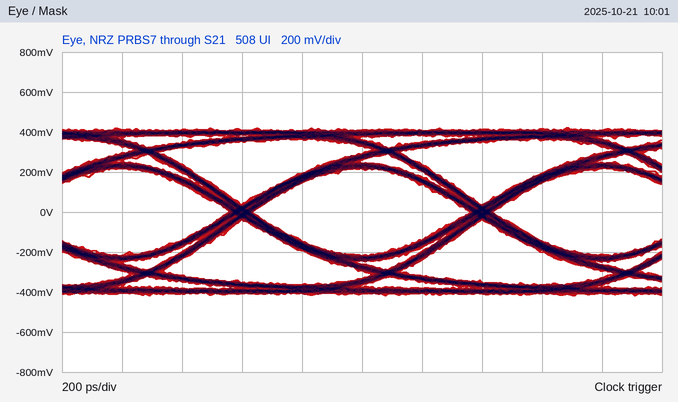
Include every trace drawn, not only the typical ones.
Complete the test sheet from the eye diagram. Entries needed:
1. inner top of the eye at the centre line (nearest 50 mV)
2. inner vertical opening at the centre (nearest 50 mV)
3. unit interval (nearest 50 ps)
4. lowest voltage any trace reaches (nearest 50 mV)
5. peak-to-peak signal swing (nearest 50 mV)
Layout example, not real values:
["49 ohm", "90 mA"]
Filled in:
["200 mV", "450 mV", "800 ps", "-400 mV", "850 mV"]
